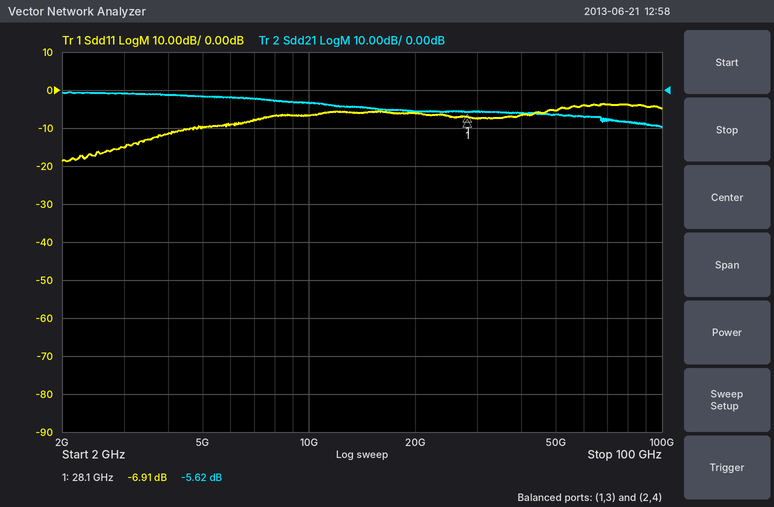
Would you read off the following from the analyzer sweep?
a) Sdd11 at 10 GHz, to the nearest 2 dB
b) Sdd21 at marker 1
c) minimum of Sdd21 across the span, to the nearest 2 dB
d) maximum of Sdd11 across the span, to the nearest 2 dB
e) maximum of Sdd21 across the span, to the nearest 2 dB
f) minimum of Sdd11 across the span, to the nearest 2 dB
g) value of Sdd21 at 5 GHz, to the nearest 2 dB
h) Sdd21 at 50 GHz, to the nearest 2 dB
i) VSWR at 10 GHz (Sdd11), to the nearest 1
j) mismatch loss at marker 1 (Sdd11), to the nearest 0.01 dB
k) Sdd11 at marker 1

-6 dB
-5.62 dB
-10 dB
-4 dB
0 dB
-18 dB
-2 dB
-6 dB
3
0.99 dB
-6.91 dB
